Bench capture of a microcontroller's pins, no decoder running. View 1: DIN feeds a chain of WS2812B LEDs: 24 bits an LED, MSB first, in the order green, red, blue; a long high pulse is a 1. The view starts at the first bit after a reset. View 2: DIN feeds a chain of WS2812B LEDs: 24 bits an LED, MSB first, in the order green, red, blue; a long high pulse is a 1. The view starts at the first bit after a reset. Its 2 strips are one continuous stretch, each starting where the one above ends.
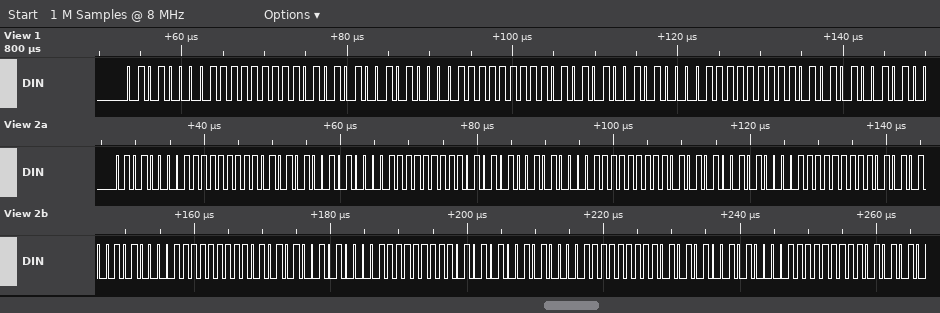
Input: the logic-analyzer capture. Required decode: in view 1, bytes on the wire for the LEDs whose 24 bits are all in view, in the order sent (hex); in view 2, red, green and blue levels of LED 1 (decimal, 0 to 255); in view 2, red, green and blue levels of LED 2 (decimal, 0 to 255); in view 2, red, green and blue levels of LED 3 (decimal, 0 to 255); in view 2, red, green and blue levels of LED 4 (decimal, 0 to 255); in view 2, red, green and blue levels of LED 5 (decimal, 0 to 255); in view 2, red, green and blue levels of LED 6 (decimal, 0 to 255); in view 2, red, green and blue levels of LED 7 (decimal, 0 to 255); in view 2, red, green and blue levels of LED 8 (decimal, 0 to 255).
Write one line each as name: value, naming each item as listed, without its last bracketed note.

in view 1, bytes on the wire for the LEDs whose 24 bits are all in view, in the order sent: 50 FF AA 50 FF AA 50 FF AA
in view 2, red, green and blue levels of LED 1: 255, 80, 170
in view 2, red, green and blue levels of LED 2: 255, 80, 170
in view 2, red, green and blue levels of LED 3: 255, 80, 170
in view 2, red, green and blue levels of LED 4: 255, 80, 170
in view 2, red, green and blue levels of LED 5: 255, 80, 170
in view 2, red, green and blue levels of LED 6: 255, 80, 170
in view 2, red, green and blue levels of LED 7: 255, 80, 170
in view 2, red, green and blue levels of LED 8: 255, 80, 170
